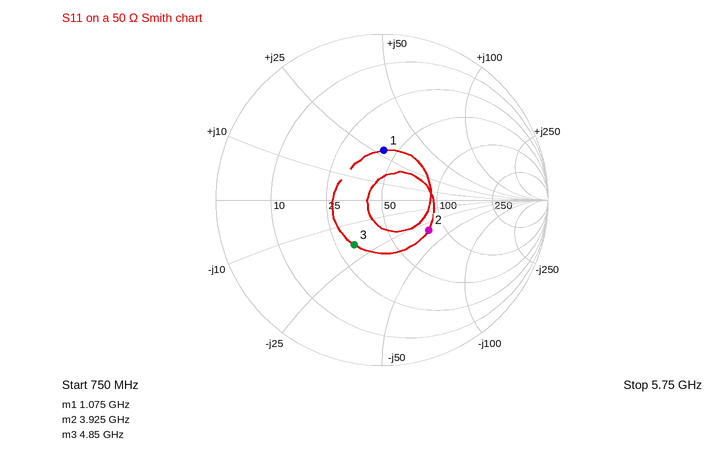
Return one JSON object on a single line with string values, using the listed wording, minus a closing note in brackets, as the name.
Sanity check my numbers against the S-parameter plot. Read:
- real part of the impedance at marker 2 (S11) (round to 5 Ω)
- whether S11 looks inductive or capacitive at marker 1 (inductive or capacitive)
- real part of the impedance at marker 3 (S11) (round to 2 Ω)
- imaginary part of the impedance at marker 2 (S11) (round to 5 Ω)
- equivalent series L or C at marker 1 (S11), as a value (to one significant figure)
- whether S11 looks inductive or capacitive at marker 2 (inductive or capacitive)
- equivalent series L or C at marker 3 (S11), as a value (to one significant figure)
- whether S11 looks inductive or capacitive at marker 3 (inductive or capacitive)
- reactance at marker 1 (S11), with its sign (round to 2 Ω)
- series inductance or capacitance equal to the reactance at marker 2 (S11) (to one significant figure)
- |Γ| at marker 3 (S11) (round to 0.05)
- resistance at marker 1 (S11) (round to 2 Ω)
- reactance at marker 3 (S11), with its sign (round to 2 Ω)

{"real part of the impedance at marker 2 (S11)": "80 Ω", "whether S11 looks inductive or capacitive at marker 1": "inductive", "real part of the impedance at marker 3 (S11)": "32 Ω", "imaginary part of the impedance at marker 2 (S11)": "-35 Ω", "equivalent series L or C at marker 1 (S11), as a value": "4 nH", "whether S11 looks inductive or capacitive at marker 2": "capacitive", "equivalent series L or C at marker 3 (S11), as a value": "2 pF", "whether S11 looks inductive or capacitive at marker 3": "capacitive", "reactance at marker 1 (S11), with its sign": "+28 Ω", "series inductance or capacitance equal to the reactance at marker 2 (S11)": "1 pF", "|Γ| at marker 3 (S11)": "0.30", "resistance at marker 1 (S11)": "42 Ω", "reactance at marker 3 (S11), with its sign": "-18 Ω"}
